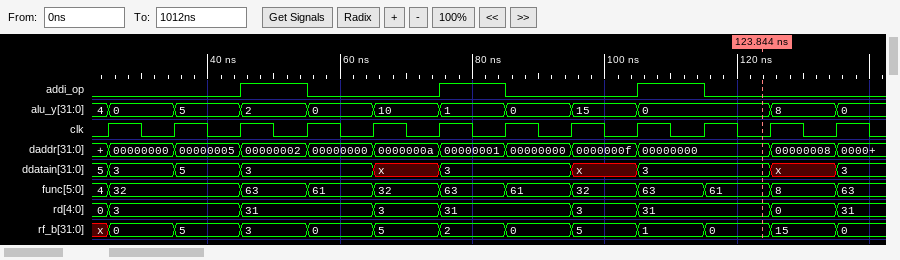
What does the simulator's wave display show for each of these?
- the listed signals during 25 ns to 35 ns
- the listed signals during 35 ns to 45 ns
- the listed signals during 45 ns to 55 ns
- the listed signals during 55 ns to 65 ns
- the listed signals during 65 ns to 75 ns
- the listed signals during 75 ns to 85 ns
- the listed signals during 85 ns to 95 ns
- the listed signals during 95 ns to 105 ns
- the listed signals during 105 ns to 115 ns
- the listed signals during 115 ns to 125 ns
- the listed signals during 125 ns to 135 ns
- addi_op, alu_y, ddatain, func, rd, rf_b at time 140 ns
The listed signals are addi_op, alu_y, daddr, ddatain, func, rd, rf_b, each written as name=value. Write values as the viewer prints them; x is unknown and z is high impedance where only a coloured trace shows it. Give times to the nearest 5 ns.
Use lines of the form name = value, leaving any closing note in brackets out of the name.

the listed signals during 25 ns to 35 ns = addi_op=0, alu_y=0, daddr=00000000, ddatain=3, func=32, rd=3, rf_b=0
the listed signals during 35 ns to 45 ns = addi_op=0, alu_y=5, daddr=00000005, ddatain=5, func=32, rd=3, rf_b=5
the listed signals during 45 ns to 55 ns = addi_op=1, alu_y=2, daddr=00000002, ddatain=3, func=63, rd=31, rf_b=3
the listed signals during 55 ns to 65 ns = addi_op=0, alu_y=0, daddr=00000000, ddatain=3, func=61, rd=31, rf_b=0
the listed signals during 65 ns to 75 ns = addi_op=0, alu_y=10, daddr=0000000a, ddatain=x, func=32, rd=3, rf_b=5
the listed signals during 75 ns to 85 ns = addi_op=1, alu_y=1, daddr=00000001, ddatain=3, func=63, rd=31, rf_b=2
the listed signals during 85 ns to 95 ns = addi_op=0, alu_y=0, daddr=00000000, ddatain=3, func=61, rd=31, rf_b=0
the listed signals during 95 ns to 105 ns = addi_op=0, alu_y=15, daddr=0000000f, ddatain=x, func=32, rd=3, rf_b=5
the listed signals during 105 ns to 115 ns = addi_op=1, alu_y=0, daddr=00000000, ddatain=3, func=63, rd=31, rf_b=1
the listed signals during 115 ns to 125 ns = addi_op=0, alu_y=0, daddr=00000000, ddatain=3, func=61, rd=31, rf_b=0
the listed signals during 125 ns to 135 ns = addi_op=0, alu_y=8, daddr=00000008, ddatain=x, func=8, rd=0, rf_b=15
addi_op, alu_y, ddatain, func, rd, rf_b at time 140 ns = addi_op=0, alu_y=0, ddatain=3, func=63, rd=31, rf_b=0
